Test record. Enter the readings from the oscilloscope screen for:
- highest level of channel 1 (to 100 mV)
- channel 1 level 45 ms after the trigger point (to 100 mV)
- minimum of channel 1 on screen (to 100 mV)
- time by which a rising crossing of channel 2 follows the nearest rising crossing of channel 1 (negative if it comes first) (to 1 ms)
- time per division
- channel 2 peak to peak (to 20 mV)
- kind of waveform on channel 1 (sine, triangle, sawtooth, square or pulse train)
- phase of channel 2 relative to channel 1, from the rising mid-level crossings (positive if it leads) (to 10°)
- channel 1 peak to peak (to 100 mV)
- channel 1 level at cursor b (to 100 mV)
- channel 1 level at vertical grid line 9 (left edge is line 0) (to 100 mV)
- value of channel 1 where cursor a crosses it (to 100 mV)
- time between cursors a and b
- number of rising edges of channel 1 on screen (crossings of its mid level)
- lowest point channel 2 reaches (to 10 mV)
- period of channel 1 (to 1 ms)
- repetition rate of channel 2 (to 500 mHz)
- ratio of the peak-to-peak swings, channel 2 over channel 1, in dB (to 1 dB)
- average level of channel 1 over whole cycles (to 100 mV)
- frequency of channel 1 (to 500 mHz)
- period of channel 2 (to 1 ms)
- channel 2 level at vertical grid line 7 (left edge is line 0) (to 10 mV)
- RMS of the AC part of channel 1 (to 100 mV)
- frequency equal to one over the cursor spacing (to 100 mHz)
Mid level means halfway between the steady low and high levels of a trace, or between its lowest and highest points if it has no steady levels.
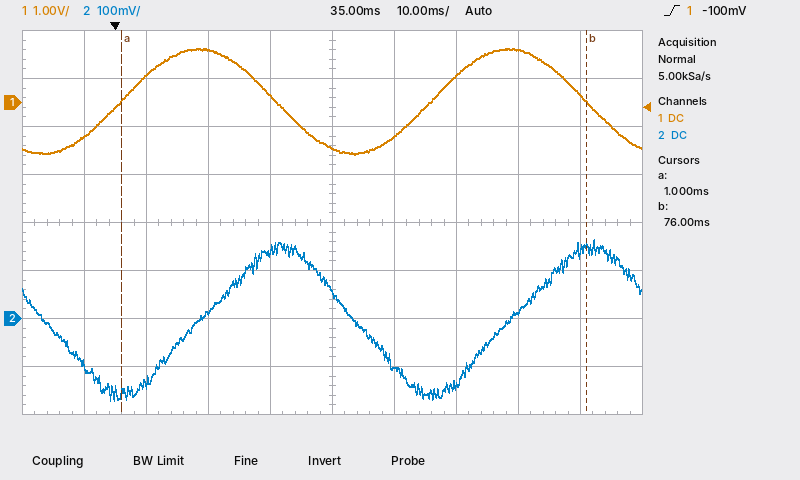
1.1 V
-700 mV
-1.1 V
+13 ms
10 ms
340 mV
sine
-90°
2.2 V
0.0 V
200 mV
0.0 V
75 ms
2
-170 mV
50 ms
20.0 Hz
-16 dB
0.0 V
20.0 Hz
50 ms
-140 mV
800 mV
13.3 Hz
